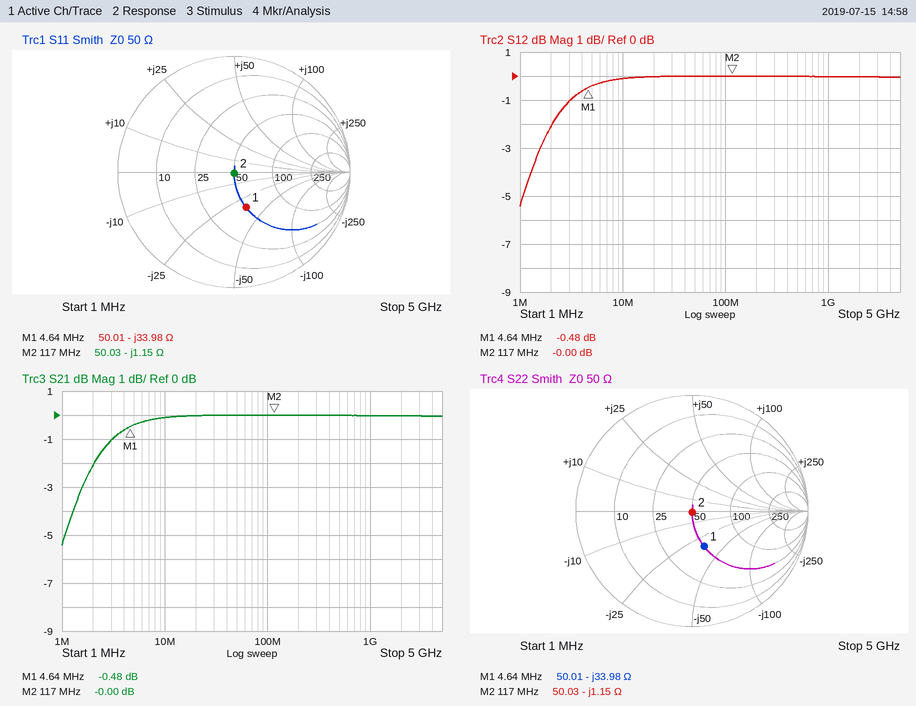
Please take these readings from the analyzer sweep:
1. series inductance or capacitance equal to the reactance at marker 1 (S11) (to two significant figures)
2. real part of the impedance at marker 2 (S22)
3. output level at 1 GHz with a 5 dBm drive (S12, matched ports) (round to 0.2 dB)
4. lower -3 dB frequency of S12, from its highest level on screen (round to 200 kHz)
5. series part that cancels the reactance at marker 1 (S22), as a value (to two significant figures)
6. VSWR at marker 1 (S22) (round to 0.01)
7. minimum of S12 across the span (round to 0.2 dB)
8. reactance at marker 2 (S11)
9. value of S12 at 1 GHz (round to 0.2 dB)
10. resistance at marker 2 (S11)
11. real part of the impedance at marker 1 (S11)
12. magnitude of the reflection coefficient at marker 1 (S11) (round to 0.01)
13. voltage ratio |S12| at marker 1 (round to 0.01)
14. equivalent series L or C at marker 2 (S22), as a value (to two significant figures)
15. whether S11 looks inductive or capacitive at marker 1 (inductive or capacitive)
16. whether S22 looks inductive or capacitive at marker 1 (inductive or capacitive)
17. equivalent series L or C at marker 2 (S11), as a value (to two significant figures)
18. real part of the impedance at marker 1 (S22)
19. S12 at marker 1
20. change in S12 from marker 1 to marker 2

1.0 nF
50.03 Ω
5.0 dBm
1.6 MHz
1.2 µH
1.95
-5.4 dB
-1.15 Ω
0.0 dB
50.03 Ω
50.01 Ω
0.32
0.95
1.2 nF
capacitive
capacitive
1.2 nF
50.01 Ω
-0.48 dB
0.48 dB
